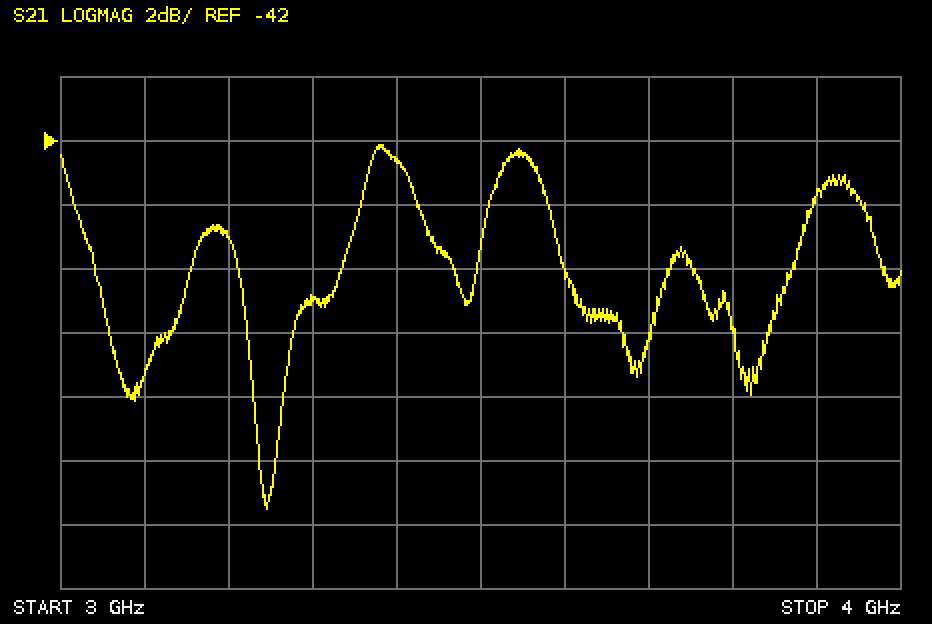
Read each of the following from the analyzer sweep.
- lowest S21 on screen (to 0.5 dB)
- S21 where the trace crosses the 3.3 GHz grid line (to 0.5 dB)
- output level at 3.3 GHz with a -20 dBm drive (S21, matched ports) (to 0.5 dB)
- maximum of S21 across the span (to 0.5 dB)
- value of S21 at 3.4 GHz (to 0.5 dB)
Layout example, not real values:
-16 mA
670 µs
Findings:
-53.5 dB
-47.0 dB
-67.0 dBm
-42.0 dB
-42.5 dB
